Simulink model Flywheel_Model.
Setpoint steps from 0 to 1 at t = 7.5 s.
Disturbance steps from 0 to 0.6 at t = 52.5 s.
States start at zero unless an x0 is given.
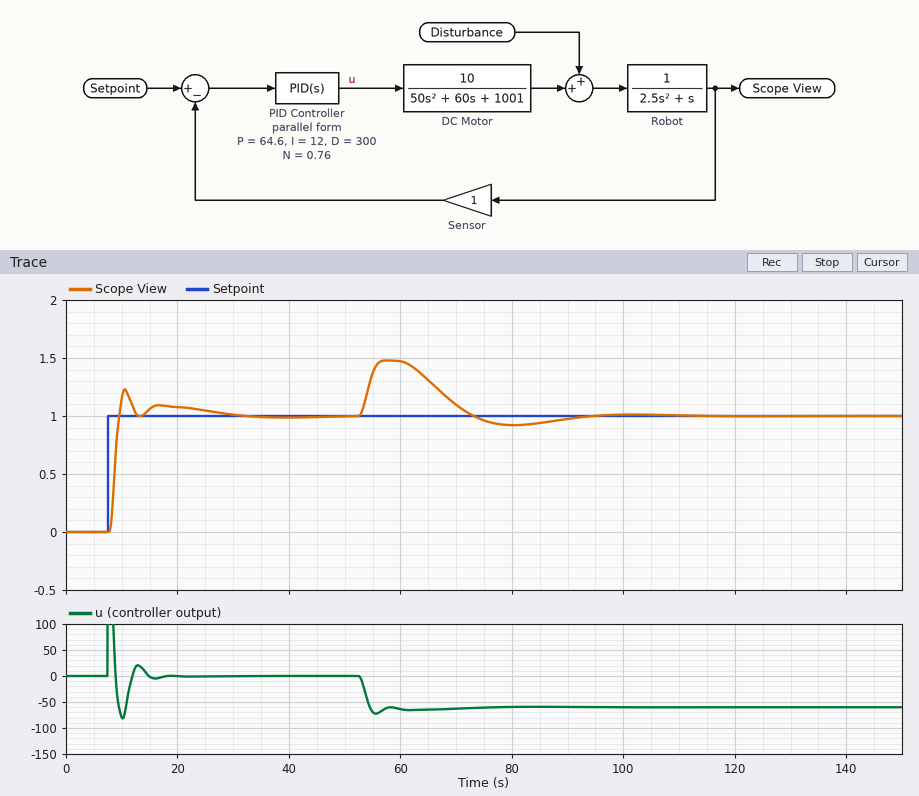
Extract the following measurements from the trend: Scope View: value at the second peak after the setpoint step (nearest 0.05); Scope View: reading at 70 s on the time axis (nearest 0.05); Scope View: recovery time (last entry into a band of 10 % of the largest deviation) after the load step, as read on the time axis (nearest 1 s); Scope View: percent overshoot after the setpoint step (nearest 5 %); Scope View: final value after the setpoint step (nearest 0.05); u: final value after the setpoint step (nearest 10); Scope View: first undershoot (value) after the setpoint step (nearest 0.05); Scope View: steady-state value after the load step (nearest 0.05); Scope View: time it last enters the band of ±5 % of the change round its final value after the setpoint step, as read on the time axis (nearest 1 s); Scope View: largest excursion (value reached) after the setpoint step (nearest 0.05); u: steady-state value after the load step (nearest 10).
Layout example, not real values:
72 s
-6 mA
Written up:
1.10
1.10
87 s
25 %
1.00
0
1.00
1.00
25 s
1.25
-60
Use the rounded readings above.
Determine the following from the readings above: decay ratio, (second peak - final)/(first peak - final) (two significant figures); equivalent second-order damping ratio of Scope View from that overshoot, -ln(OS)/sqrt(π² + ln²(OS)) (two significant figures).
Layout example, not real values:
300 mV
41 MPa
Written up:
0.40
0.40
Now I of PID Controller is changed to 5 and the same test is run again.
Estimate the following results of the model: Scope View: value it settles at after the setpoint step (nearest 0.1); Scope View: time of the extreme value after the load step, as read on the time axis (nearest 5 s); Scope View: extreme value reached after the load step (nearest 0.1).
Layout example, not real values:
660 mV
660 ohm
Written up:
1.0
60 s
1.6
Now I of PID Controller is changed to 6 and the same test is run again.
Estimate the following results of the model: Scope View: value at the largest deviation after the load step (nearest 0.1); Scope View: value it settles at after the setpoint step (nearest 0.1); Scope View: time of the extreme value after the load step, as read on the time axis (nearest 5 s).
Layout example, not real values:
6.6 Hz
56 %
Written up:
1.6
1.0
60 s
